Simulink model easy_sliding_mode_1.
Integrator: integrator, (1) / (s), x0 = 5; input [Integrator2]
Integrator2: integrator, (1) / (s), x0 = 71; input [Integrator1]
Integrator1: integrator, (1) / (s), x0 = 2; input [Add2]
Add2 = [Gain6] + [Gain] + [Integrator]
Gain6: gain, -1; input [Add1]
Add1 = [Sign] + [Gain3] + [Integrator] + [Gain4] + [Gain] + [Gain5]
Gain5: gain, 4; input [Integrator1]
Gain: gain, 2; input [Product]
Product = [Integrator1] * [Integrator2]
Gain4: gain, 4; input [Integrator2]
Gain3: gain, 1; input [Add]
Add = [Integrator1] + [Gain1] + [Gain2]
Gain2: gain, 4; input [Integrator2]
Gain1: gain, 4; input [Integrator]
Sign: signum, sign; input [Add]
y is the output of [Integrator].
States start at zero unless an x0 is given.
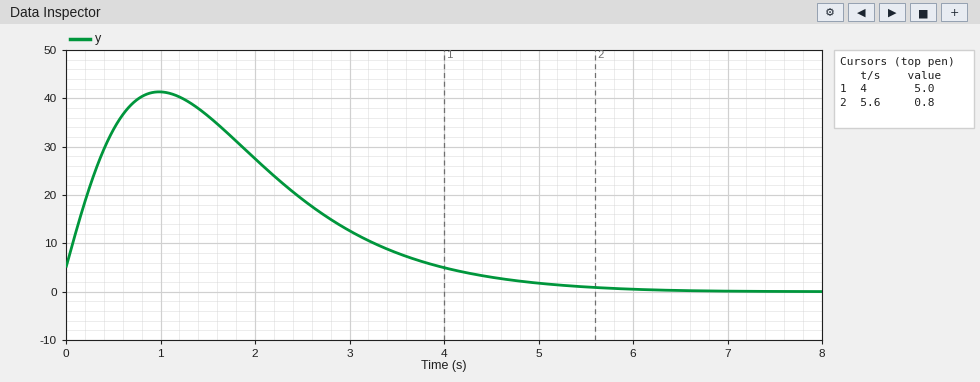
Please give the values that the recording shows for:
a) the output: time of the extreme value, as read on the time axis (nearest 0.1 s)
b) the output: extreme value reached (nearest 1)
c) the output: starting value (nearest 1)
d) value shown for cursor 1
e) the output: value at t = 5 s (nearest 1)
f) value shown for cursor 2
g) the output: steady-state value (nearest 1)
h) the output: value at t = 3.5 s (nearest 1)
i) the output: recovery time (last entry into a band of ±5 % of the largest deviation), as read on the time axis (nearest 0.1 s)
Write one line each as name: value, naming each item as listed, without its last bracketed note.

the output: time of the extreme value, as read on the time axis: 1.0 s
the output: extreme value reached: 41
the output: starting value: 5
value shown for cursor 1: 5.0
the output: value at t = 5 s: 2
value shown for cursor 2: 0.8
the output: steady-state value: 0
the output: value at t = 3.5 s: 8
the output: recovery time (last entry into a band of ±5 % of the largest deviation), as read on the time axis: 5.0 s
